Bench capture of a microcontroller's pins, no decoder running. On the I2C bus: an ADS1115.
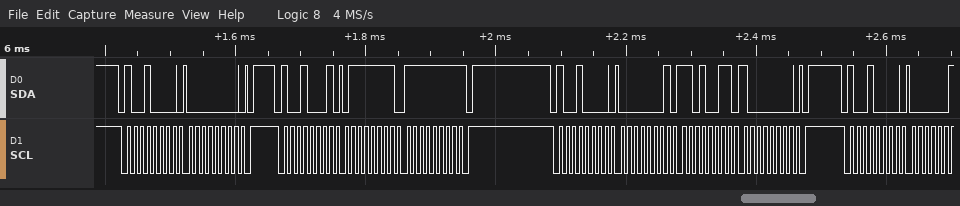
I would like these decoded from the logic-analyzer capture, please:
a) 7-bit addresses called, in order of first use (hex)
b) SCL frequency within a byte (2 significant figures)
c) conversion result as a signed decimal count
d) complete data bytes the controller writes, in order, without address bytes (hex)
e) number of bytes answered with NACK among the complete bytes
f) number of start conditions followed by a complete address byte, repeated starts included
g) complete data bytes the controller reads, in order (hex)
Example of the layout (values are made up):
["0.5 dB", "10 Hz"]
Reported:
["0x48", "100 kHz", "32767", "00 01 D3 80", "1", "4", "7F FF"]
